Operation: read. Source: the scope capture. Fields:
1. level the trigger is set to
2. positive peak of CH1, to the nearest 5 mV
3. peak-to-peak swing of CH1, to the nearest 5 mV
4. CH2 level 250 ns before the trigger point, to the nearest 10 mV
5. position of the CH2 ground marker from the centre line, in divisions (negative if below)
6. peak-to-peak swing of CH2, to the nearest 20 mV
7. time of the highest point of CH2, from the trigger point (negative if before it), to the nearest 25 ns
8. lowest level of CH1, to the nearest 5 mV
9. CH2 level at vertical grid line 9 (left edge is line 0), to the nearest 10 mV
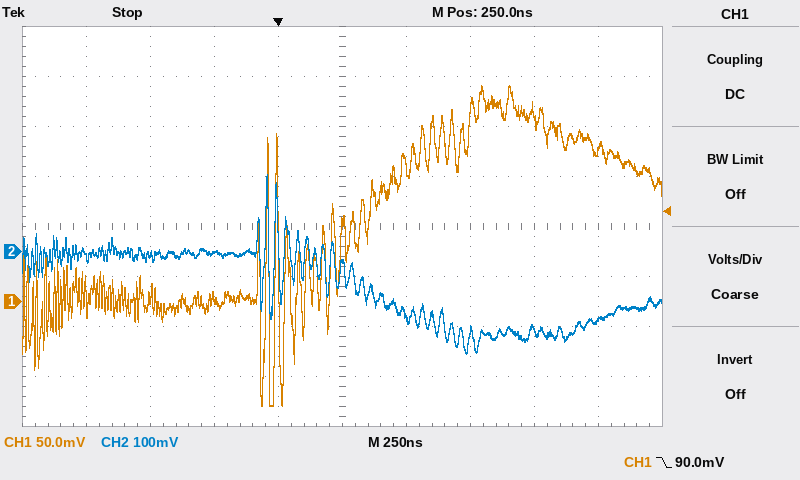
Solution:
90.0 mV
215 mV
320 mV
0 mV
-0.5 div
360 mV
-50 ns
-105 mV
-140 mV
